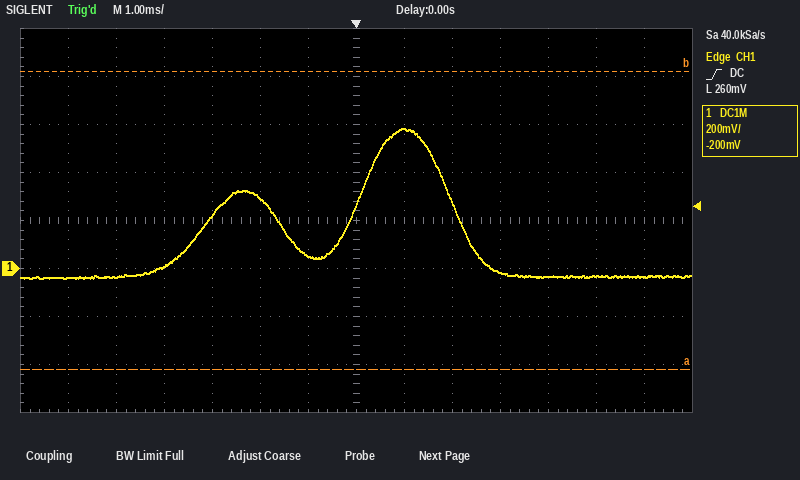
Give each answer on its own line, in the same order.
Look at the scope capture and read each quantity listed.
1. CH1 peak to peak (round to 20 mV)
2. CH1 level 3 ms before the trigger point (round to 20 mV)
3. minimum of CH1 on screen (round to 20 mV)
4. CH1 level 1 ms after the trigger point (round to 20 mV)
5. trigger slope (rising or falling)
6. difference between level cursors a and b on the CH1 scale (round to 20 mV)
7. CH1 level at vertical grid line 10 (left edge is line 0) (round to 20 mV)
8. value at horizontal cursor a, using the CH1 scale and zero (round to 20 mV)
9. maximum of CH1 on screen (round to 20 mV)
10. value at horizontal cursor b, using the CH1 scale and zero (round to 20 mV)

620 mV
220 mV
-40 mV
580 mV
rising
1.24 V
-20 mV
-420 mV
580 mV
820 mV
